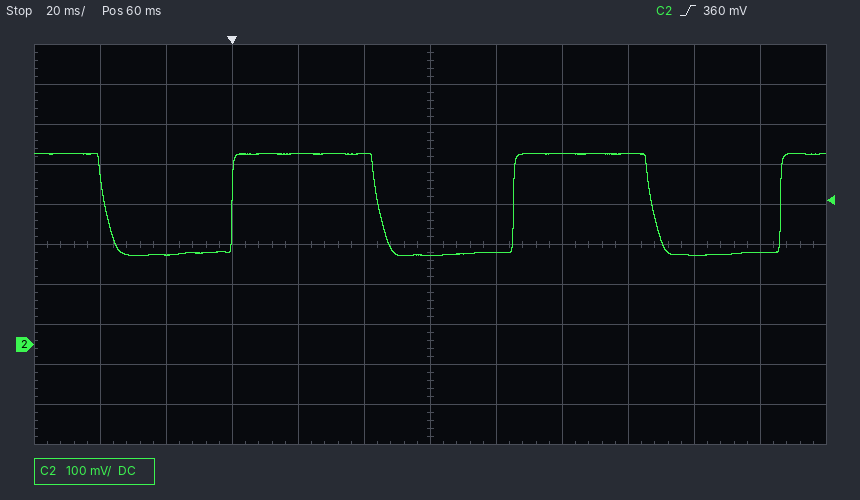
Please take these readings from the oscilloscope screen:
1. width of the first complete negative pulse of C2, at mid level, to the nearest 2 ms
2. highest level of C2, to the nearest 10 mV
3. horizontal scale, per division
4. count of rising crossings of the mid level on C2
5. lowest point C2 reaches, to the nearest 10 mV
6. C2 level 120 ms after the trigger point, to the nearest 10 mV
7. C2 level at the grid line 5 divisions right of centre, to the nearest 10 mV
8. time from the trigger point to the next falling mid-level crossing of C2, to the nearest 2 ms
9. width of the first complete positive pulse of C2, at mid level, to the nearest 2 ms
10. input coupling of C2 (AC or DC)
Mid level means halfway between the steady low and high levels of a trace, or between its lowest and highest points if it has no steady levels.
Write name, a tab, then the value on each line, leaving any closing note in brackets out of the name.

width of the first complete negative pulse of C2, at mid level, to the nearest 2 ms	38 ms
highest level of C2, to the nearest 10 mV	480 mV
horizontal scale, per division	20 ms
count of rising crossings of the mid level on C2	3
lowest point C2 reaches, to the nearest 10 mV	220 mV
C2 level 120 ms after the trigger point, to the nearest 10 mV	480 mV
C2 level at the grid line 5 divisions right of centre, to the nearest 10 mV	230 mV
time from the trigger point to the next falling mid-level crossing of C2, to the nearest 2 ms	44 ms
width of the first complete positive pulse of C2, at mid level, to the nearest 2 ms	44 ms
input coupling of C2	DC
